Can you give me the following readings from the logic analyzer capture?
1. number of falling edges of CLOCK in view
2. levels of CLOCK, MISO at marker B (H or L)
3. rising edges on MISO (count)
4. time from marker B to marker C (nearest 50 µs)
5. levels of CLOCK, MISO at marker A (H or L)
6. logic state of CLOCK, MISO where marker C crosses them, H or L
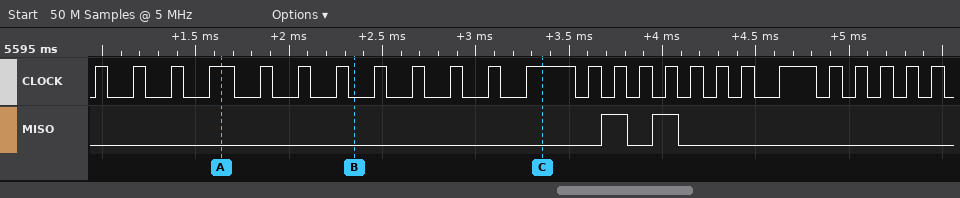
25
CLOCK=L, MISO=L
2
1000 µs
CLOCK=H, MISO=L
CLOCK=H, MISO=L
